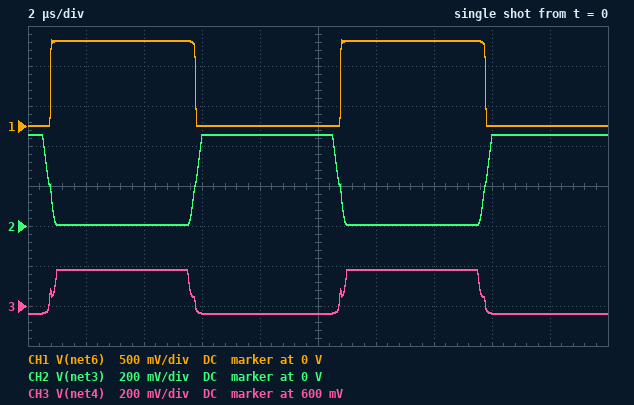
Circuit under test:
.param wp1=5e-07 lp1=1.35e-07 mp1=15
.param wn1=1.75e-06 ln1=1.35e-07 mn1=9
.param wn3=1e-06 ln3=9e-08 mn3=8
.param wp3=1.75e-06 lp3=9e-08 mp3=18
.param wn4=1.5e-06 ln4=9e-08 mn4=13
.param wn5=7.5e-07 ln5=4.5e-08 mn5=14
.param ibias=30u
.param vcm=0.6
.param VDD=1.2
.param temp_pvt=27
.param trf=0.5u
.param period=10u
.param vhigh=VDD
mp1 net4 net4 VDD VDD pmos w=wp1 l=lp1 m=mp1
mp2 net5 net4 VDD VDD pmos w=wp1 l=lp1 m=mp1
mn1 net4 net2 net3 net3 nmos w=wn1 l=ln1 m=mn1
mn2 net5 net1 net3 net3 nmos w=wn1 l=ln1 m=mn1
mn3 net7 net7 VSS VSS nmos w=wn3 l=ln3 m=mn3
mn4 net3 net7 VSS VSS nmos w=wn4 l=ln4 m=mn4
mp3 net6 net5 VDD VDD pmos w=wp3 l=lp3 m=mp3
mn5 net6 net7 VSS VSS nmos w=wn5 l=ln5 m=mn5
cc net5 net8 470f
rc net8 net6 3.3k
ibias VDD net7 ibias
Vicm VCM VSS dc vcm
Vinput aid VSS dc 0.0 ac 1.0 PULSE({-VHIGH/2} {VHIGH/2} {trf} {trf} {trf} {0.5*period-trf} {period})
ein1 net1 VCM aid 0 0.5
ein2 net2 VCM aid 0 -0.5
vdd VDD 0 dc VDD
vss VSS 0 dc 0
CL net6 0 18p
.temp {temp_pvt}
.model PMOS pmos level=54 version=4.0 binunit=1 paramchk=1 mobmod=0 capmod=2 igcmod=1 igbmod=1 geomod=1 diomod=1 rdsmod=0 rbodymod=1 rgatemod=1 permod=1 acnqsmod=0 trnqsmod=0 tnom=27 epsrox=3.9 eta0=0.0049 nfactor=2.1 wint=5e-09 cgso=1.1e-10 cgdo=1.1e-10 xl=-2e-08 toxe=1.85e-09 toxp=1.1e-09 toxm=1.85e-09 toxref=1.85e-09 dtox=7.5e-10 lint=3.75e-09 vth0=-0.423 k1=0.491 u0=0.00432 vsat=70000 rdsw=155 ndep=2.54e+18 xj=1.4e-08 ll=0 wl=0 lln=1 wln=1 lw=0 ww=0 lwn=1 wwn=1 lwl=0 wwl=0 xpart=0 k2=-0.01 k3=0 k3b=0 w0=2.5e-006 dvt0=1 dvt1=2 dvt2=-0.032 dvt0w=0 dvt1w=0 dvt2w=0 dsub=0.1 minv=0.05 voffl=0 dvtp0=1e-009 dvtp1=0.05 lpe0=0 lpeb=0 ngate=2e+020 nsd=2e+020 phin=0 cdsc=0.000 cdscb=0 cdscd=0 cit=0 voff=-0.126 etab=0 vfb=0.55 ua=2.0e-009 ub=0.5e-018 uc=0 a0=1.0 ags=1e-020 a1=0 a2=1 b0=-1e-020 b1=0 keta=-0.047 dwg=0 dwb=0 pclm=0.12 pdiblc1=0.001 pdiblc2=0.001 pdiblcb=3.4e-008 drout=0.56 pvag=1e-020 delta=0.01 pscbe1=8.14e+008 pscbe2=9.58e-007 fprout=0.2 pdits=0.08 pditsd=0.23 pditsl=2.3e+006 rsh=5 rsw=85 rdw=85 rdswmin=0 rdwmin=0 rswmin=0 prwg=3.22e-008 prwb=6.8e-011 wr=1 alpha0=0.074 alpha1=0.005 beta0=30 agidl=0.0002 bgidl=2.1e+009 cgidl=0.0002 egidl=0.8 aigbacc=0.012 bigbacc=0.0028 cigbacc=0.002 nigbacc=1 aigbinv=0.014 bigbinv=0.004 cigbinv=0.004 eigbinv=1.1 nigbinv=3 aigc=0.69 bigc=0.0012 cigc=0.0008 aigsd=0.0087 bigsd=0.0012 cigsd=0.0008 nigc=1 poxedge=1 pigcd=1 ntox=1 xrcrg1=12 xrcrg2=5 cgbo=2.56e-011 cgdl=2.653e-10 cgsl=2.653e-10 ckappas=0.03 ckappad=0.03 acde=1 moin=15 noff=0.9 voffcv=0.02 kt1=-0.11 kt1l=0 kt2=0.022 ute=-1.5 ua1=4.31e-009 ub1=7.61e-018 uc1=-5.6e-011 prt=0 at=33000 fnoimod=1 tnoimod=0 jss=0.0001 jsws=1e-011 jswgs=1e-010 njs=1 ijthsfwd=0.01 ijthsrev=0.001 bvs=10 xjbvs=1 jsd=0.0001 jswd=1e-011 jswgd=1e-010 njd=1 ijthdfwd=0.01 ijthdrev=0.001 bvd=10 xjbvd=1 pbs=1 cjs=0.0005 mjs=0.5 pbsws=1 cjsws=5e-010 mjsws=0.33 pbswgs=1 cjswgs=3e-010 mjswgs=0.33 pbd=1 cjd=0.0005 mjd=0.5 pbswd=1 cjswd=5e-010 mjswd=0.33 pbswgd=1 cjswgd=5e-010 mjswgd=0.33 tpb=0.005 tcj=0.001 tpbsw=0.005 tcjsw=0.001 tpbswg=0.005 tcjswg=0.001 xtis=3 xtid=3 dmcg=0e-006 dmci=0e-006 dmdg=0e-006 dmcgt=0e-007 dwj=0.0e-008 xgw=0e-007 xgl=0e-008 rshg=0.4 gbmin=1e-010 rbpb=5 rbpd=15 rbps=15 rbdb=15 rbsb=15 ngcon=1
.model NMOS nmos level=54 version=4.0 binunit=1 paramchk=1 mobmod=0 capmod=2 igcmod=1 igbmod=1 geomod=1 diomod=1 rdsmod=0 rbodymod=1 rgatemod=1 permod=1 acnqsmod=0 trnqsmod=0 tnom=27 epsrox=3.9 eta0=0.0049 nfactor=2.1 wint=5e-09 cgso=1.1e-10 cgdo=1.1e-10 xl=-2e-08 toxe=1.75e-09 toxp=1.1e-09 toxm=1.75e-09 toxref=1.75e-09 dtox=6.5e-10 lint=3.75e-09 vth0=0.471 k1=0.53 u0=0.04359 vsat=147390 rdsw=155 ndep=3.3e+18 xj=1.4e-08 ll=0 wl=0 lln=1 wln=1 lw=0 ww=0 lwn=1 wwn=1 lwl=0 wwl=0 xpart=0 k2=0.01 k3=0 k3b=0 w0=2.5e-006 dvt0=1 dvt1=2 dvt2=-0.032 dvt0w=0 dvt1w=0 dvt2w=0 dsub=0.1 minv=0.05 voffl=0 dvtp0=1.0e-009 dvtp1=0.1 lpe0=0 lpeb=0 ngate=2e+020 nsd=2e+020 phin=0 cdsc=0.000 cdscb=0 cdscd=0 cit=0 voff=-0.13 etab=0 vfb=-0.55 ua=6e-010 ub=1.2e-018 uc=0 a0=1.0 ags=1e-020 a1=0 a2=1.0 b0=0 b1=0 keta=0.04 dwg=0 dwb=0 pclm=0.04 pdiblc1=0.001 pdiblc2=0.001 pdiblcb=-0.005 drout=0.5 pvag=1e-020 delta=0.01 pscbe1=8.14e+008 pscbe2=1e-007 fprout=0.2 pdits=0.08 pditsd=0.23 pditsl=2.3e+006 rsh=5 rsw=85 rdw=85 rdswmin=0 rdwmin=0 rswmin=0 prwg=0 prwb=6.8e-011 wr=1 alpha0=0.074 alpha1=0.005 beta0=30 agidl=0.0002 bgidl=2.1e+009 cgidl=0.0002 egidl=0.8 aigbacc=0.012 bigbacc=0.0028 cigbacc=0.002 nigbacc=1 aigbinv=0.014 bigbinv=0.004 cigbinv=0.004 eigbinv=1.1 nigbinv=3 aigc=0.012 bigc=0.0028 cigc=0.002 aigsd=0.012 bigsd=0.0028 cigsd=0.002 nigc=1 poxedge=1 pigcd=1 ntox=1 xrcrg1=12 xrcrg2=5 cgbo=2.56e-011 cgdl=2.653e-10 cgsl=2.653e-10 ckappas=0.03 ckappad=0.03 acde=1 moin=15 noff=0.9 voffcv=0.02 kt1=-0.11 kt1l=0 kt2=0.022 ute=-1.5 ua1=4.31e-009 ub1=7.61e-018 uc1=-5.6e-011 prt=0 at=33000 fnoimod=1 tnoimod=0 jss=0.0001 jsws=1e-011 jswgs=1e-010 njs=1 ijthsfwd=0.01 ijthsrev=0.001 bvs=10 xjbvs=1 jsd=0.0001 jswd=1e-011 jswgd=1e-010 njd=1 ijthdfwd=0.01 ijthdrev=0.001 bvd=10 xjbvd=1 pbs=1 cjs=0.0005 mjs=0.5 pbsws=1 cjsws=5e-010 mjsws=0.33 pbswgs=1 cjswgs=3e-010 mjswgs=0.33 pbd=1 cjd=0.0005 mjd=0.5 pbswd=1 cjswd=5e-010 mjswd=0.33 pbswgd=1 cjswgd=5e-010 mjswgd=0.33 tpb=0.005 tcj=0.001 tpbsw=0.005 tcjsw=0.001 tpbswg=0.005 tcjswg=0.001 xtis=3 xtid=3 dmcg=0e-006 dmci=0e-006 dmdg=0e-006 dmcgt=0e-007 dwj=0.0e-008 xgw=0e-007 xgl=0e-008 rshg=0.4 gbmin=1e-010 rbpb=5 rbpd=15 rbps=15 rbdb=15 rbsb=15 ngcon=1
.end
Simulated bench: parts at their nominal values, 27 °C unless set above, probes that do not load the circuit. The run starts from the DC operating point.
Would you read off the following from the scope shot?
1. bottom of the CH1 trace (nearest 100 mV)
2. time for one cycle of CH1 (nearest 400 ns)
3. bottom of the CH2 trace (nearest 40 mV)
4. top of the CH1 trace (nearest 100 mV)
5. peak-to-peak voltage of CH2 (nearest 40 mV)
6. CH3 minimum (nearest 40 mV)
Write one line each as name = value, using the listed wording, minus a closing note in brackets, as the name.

bottom of the CH1 trace = 0 V
time for one cycle of CH1 = 10.0 µs
bottom of the CH2 trace = 0 V
top of the CH1 trace = 1.1 V
peak-to-peak voltage of CH2 = 440 mV
CH3 minimum = 560 mV
